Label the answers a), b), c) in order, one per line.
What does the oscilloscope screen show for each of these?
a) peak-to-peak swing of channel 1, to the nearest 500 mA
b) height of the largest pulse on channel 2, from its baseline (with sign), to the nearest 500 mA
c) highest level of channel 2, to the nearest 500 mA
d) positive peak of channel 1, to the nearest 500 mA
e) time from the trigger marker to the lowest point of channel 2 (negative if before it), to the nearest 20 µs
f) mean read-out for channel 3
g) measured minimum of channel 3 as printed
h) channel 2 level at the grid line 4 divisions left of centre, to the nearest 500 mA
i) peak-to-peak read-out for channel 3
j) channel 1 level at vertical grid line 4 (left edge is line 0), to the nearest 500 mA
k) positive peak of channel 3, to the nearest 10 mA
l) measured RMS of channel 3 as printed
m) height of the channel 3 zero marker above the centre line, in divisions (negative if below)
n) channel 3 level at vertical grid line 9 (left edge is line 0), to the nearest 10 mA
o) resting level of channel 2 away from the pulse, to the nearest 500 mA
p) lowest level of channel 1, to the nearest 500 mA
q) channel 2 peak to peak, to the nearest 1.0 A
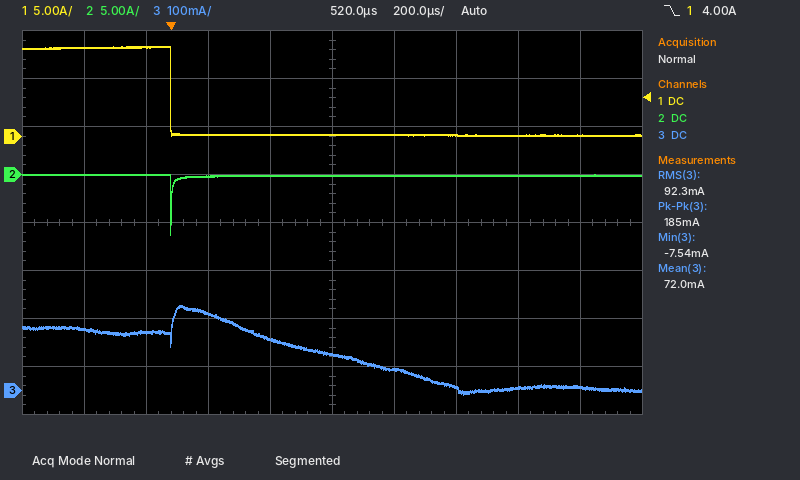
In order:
a) 9.5 A
b) -6.0 A
c) 0.0 A
d) 9.5 A
e) 0 µs
f) 72.0 mA
g) -7.54 mA
h) 0.0 A
i) 185 mA
j) 0.0 A
k) 180 mA
l) 92.3 mA
m) -3.5 div
n) 10 mA
o) 0.0 A
p) 0.0 A
q) 6.0 A
